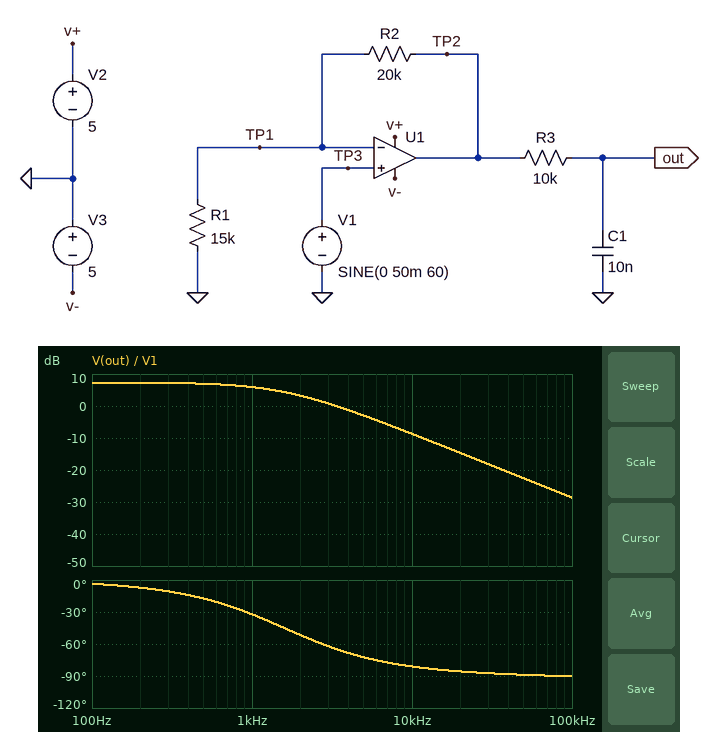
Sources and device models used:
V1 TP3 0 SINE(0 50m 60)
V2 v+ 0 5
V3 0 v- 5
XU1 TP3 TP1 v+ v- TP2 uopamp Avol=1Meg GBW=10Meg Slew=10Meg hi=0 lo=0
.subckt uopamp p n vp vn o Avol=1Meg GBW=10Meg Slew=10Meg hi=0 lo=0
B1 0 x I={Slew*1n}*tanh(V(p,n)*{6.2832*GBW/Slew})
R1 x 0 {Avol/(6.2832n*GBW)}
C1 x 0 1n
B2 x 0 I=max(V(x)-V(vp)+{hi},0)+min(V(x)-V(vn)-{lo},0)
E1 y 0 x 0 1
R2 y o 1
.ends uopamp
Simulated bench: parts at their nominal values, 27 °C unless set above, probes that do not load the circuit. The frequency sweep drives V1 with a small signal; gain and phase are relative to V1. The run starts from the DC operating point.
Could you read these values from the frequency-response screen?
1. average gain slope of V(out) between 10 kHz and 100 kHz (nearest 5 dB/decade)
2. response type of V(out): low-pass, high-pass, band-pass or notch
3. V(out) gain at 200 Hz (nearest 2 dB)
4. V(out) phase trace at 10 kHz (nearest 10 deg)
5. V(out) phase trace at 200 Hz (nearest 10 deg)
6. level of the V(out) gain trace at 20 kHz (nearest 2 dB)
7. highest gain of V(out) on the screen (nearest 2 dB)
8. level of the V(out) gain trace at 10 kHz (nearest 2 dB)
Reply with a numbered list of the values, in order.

1. -20 dB/decade
2. low-pass
3. 8 dB
4. -80 deg
5. -10 deg
6. -14 dB
7. 8 dB
8. -8 dB
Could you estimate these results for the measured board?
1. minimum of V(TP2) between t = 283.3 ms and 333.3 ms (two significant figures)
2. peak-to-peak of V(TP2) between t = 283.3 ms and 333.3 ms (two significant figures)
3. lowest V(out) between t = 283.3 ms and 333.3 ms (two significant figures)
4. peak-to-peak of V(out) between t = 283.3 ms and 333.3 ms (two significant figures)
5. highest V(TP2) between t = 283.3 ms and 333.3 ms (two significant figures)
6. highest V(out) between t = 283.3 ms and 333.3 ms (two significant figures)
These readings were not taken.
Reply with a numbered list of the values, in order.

1. -120 mV
2. 230 mV
3. -120 mV
4. 230 mV
5. 120 mV
6. 120 mV
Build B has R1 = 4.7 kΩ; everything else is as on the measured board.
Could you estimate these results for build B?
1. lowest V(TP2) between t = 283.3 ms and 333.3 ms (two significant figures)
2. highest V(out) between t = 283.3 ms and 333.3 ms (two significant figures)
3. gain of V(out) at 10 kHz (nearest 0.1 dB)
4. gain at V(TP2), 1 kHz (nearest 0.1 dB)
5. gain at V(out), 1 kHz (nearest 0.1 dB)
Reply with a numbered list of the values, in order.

1. -260 mV
2. 260 mV
3. -1.7 dB
4. 14.4 dB
5. 13.0 dB
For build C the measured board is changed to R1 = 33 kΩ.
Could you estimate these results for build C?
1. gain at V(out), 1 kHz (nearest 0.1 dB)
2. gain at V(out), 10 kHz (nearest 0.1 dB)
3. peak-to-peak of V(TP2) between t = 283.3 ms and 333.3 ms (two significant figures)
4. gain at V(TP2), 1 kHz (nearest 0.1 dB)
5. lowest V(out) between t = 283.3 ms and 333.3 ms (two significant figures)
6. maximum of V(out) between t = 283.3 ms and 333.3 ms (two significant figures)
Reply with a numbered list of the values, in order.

1. 2.7 dB
2. -12.0 dB
3. 160 mV
4. 4.1 dB
5. -80 mV
6. 80 mV
